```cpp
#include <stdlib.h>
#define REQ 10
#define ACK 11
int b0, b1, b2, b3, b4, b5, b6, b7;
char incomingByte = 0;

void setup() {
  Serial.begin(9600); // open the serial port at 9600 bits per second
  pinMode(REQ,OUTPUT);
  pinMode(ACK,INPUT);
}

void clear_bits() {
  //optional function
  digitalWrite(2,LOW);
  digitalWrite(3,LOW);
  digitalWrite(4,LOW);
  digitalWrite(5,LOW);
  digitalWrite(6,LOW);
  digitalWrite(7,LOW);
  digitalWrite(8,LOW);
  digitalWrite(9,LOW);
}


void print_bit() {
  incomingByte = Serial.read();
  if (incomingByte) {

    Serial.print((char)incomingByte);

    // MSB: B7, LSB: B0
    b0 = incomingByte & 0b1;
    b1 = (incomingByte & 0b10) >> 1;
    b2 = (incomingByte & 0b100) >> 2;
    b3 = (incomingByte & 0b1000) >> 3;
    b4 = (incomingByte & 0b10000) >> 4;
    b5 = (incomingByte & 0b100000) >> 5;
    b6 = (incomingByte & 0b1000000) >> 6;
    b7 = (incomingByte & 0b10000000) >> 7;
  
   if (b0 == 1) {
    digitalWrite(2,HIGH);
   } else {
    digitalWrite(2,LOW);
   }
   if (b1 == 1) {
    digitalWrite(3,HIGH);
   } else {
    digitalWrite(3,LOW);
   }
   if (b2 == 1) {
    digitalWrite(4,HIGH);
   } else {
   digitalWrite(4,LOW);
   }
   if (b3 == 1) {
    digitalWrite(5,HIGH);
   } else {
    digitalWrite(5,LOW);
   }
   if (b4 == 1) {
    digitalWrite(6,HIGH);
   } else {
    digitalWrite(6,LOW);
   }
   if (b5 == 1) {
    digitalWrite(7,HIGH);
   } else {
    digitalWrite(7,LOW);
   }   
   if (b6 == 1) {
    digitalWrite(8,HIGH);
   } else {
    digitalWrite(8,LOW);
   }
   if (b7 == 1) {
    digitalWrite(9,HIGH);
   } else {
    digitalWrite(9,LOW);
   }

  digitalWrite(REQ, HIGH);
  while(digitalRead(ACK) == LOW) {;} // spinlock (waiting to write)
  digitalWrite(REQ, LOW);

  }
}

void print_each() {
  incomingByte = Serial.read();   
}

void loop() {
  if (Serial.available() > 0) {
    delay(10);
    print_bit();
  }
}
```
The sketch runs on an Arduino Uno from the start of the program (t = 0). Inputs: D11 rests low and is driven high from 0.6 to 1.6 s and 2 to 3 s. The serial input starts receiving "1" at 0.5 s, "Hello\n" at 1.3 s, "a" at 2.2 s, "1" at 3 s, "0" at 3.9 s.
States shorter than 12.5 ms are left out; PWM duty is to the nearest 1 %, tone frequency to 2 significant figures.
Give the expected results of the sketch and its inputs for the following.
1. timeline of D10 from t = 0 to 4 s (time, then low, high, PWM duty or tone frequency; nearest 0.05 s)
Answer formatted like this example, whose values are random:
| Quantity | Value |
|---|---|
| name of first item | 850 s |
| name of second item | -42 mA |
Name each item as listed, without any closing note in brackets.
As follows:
| Quantity | Value |
|---|---|
| timeline of D10 from t = 0 to 4 s | 0 s low; 0.5 s high; 0.6 s low; 1.3 s tone 110 Hz; 1.35 s low; 3 s high |
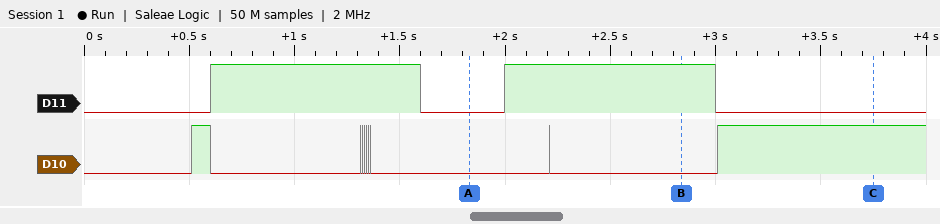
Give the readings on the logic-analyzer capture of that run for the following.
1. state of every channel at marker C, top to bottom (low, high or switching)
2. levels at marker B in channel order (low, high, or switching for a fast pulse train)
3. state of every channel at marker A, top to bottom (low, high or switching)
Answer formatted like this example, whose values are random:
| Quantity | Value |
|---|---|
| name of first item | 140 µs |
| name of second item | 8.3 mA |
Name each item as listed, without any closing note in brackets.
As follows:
| Quantity | Value |
|---|---|
| state of every channel at marker C, top to bottom | D11 low, D10 high |
| levels at marker B in channel order | D11 high, D10 low |
| state of every channel at marker A, top to bottom | D11 low, D10 low |
